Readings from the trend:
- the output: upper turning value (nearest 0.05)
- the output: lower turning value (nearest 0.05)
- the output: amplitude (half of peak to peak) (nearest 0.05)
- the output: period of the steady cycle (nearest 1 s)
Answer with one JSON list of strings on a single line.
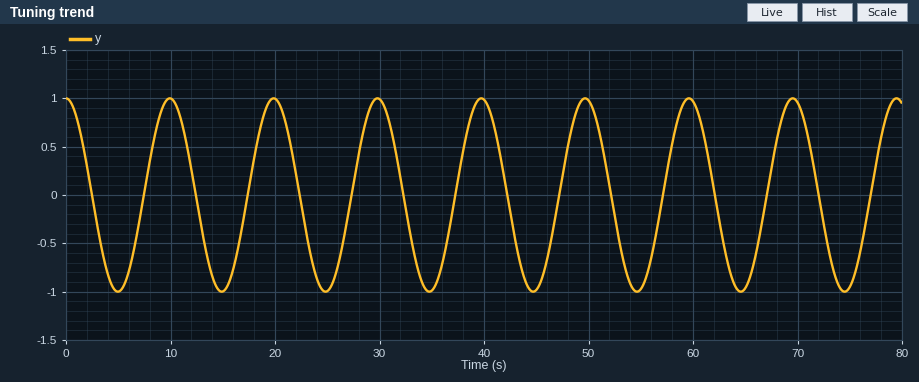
["1.00", "-1.00", "1.00", "10 s"]
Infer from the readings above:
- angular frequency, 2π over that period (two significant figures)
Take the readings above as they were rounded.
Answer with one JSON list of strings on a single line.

["0.63 rad/s"]
